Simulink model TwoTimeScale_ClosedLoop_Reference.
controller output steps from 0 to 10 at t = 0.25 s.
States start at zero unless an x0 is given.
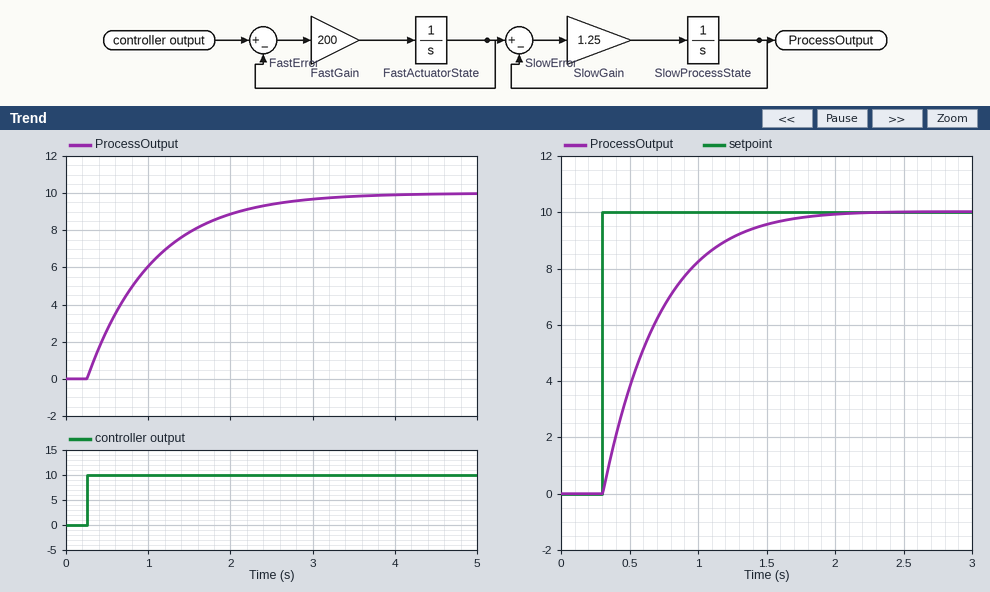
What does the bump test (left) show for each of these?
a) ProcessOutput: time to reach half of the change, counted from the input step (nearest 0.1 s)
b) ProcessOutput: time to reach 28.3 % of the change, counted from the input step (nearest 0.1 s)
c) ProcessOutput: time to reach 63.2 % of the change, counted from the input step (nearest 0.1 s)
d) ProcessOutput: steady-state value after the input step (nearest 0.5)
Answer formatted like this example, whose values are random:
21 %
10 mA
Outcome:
0.6 s
0.3 s
0.8 s
10.0
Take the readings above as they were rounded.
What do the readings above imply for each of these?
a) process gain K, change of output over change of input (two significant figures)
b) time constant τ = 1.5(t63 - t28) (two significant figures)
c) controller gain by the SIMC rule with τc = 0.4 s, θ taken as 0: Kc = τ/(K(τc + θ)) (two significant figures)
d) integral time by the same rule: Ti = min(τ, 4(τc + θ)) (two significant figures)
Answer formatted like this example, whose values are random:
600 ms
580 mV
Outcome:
1.0
0.75 s
1.9
0.75 s
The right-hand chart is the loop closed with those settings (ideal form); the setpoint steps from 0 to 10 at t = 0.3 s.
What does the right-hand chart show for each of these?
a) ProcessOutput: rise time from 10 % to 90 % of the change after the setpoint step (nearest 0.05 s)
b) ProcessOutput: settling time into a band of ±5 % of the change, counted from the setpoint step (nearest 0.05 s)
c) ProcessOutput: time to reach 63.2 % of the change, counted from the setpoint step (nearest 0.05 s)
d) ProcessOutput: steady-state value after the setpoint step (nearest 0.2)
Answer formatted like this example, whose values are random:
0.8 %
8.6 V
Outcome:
0.85 s
1.15 s
0.40 s
10.0
